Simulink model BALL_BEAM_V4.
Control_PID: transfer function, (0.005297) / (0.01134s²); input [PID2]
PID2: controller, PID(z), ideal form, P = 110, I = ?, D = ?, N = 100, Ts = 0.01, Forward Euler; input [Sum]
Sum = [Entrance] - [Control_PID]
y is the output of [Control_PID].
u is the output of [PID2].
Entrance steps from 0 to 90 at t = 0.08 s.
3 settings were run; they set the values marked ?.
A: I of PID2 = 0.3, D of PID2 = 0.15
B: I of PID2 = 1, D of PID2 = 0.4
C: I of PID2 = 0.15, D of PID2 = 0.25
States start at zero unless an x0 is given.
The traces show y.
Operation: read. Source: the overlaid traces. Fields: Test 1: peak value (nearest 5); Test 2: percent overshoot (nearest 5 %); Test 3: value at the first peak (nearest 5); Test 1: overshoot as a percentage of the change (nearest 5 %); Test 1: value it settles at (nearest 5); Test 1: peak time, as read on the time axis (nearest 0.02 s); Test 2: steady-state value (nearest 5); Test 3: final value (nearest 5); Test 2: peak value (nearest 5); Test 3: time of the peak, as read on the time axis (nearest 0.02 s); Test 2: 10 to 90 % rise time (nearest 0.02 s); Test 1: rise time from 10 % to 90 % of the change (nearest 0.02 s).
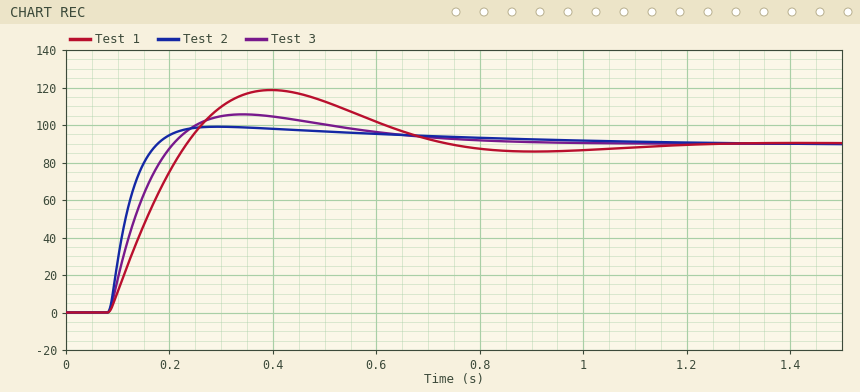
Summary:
120
10 %
105
30 %
90
0.40 s
90
90
100
0.34 s
0.06 s
0.12 s
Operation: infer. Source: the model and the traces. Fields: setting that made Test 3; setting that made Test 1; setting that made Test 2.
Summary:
C
A
B
